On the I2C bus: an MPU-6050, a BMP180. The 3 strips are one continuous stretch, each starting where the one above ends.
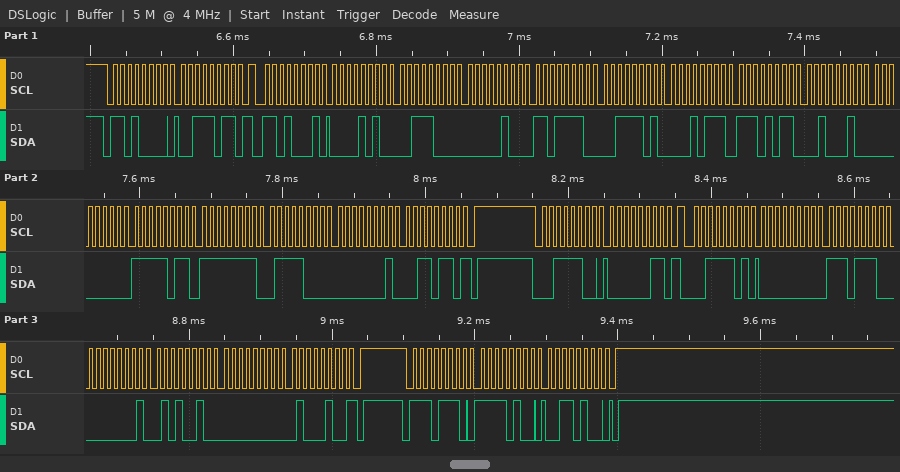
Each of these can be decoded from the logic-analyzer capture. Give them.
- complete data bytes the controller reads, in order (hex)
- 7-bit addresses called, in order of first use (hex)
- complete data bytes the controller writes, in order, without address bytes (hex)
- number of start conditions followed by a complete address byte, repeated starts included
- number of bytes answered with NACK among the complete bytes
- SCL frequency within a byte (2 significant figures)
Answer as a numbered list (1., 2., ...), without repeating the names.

1. 0A 38 04 DE 3D 17 EB 22 00 FB FF 78 01 36 00 EE 01 52 00 44
2. 0x68 0x1E 0x77
3. 3B 03 F4 34
4. 5
5. 2
6. 100 kHz
